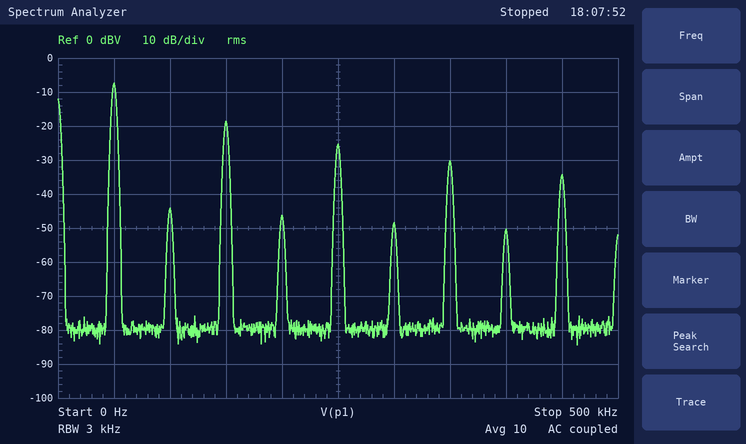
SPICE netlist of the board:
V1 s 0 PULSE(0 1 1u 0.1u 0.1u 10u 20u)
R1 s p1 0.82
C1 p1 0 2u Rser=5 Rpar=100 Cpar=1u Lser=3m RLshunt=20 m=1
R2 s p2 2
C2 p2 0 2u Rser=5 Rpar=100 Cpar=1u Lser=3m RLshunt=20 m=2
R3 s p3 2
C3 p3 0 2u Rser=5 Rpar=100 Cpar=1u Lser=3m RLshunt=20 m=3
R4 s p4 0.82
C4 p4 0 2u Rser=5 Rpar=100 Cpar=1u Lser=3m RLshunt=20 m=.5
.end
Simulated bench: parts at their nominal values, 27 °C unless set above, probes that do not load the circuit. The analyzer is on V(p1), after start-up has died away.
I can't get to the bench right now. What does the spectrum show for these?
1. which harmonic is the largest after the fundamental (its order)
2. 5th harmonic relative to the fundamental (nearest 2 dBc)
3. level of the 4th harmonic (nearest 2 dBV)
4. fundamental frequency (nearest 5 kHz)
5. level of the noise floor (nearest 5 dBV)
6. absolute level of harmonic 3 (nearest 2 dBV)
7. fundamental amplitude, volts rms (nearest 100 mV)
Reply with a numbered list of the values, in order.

1. 3
2. -18 dBc
3. -46 dBV
4. 50 kHz
5. -80 dBV
6. -18 dBV
7. 400 mV
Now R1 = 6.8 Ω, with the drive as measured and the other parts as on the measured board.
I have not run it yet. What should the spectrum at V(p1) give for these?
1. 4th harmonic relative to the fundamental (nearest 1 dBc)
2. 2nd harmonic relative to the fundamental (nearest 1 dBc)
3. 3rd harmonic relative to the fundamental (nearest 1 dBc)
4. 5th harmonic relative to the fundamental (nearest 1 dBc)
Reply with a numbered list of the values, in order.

1. -47 dBc
2. -41 dBc
3. -18 dBc
4. -27 dBc
